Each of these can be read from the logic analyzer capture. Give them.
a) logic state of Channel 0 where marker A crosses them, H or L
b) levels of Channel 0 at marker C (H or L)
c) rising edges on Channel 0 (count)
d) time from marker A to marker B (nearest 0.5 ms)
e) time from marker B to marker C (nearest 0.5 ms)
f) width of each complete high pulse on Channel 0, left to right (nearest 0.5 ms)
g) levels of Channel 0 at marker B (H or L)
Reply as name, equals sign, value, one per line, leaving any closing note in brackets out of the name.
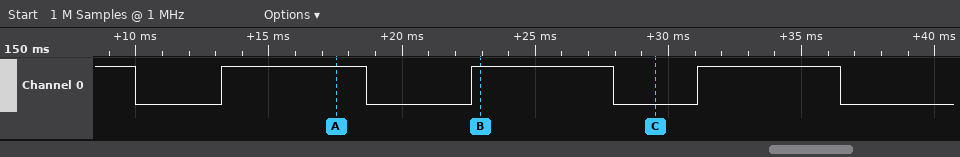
logic state of Channel 0 where marker A crosses them, H or L = Channel 0=H
levels of Channel 0 at marker C = Channel 0=L
rising edges on Channel 0 = 3
time from marker A to marker B = 5.5 ms
time from marker B to marker C = 6.5 ms
width of each complete high pulse on Channel 0, left to right = 5.5 ms, 5.5 ms, 5.5 ms
levels of Channel 0 at marker B = Channel 0=H
